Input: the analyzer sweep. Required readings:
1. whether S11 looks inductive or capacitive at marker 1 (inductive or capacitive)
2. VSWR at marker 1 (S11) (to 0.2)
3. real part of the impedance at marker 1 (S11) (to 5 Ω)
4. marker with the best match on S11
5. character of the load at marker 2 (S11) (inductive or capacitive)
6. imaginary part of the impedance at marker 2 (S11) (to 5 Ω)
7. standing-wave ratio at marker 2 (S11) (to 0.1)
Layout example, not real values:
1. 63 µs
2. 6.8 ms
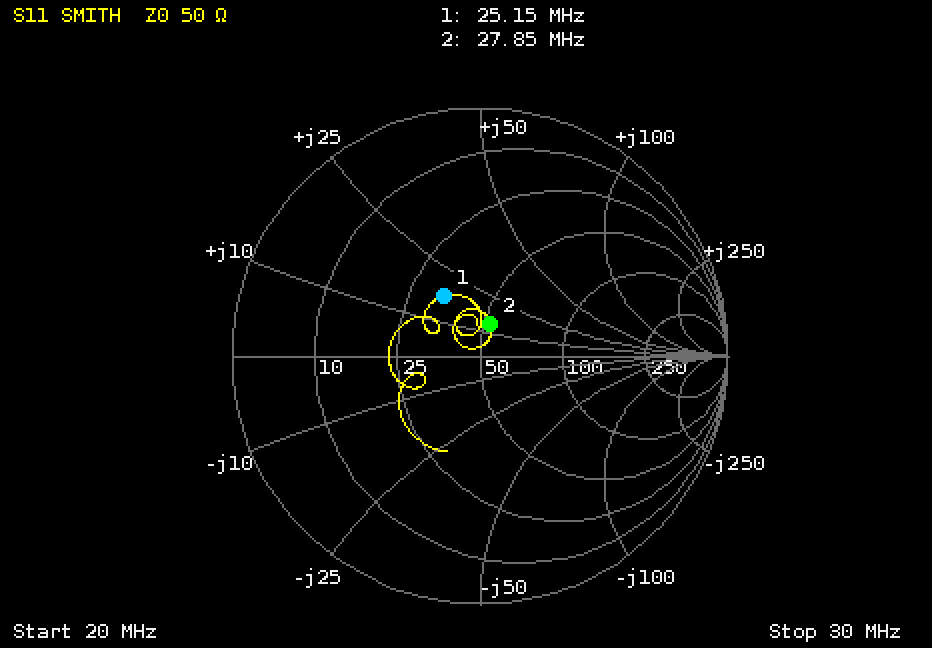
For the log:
1. inductive
2. 1.8
3. 35 Ω
4. marker 2
5. inductive
6. +15 Ω
7. 1.3
